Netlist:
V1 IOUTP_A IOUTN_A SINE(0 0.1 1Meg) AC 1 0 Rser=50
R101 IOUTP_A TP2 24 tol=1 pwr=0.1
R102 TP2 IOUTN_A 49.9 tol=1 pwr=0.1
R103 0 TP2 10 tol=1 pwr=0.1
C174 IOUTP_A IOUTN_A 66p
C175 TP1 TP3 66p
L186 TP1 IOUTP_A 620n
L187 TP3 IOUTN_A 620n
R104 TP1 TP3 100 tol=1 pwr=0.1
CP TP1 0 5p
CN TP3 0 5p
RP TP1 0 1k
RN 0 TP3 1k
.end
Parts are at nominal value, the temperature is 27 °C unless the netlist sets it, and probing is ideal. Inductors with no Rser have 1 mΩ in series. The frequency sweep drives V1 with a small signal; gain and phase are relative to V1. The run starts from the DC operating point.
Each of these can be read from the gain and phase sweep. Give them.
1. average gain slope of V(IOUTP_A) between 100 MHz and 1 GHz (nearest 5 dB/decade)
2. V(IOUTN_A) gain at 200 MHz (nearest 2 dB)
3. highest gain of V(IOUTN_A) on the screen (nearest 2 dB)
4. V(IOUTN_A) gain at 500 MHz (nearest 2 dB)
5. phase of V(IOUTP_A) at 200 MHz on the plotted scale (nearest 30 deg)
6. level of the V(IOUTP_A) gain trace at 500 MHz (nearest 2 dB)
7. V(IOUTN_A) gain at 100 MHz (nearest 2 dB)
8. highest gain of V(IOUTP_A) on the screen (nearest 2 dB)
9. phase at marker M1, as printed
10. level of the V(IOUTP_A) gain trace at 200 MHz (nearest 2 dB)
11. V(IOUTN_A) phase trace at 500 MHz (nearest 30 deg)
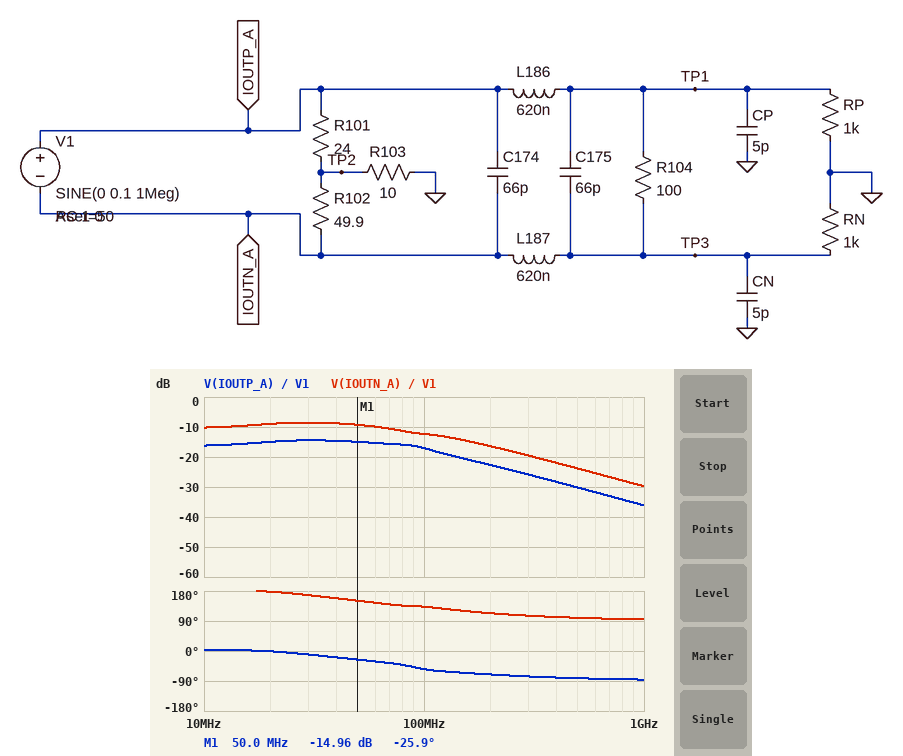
-20 dB/decade
-16 dB
-8 dB
-24 dB
-60 deg
-30 dB
-12 dB
-14 dB
-25.9 deg
-22 dB
90 deg
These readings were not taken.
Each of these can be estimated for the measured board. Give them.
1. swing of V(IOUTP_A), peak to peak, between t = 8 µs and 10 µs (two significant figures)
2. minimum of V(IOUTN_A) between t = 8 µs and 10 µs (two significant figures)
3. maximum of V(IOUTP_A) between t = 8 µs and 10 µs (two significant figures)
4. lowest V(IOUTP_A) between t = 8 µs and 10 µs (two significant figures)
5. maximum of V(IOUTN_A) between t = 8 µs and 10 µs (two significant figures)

30 mV
-30 mV
15 mV
-15 mV
30 mV
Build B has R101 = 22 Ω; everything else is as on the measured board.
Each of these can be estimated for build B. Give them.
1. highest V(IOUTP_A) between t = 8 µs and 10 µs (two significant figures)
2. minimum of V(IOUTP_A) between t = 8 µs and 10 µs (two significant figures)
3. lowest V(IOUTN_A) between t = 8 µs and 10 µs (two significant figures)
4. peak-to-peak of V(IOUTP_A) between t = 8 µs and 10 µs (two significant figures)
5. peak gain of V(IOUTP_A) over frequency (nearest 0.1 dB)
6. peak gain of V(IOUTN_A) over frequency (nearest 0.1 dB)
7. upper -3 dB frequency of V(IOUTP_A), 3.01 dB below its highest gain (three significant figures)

14 mV
-14 mV
-31 mV
28 mV
-15.0 dB
-8.4 dB
106 MHz
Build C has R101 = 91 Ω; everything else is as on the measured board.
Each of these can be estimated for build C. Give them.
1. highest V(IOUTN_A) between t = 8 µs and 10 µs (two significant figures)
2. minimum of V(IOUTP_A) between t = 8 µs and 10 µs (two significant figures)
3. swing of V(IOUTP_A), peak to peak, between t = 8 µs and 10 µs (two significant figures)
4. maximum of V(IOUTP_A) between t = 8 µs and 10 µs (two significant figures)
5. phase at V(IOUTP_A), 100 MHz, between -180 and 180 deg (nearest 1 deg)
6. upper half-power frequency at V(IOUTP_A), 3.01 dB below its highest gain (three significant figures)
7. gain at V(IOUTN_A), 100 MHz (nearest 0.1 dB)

19 mV
-34 mV
67 mV
34 mV
-53 deg
72.3 MHz
-15.5 dB
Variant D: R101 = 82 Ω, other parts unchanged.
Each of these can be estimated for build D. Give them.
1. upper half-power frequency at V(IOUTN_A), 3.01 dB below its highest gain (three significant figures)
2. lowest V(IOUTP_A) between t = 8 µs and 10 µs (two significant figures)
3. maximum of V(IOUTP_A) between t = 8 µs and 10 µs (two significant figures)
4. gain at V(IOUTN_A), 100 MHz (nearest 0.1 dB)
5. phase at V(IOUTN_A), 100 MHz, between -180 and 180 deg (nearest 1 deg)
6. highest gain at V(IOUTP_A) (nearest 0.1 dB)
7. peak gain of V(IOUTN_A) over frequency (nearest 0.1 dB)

91.7 MHz
-32 mV
32 mV
-15.2 dB
121 deg
-7.7 dB
-11.6 dB
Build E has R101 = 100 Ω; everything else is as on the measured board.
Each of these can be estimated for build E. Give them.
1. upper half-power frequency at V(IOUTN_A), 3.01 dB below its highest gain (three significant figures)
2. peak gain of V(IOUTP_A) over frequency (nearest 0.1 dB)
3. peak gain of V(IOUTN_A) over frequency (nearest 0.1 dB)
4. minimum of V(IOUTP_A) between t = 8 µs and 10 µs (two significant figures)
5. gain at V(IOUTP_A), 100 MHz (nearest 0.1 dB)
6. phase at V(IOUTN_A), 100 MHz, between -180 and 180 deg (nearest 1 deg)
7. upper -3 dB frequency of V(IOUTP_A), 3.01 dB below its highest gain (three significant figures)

95.3 MHz
-6.9 dB
-12.3 dB
-35 mV
-12.0 dB
119 deg
71.0 MHz
